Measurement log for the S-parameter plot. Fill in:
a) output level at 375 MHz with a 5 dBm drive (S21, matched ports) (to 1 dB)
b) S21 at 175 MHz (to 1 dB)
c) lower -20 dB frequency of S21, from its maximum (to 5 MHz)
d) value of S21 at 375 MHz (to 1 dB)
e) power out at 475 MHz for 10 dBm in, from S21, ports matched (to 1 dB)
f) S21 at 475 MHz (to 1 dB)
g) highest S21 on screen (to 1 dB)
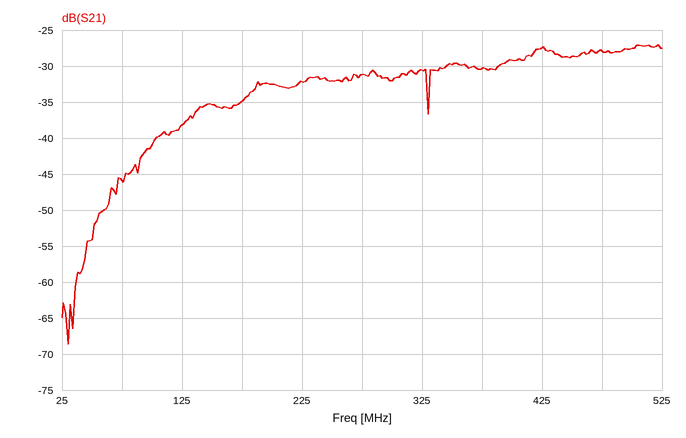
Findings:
-25 dBm
-35 dB
70 MHz
-30 dB
-18 dBm
-28 dB
-27 dB
